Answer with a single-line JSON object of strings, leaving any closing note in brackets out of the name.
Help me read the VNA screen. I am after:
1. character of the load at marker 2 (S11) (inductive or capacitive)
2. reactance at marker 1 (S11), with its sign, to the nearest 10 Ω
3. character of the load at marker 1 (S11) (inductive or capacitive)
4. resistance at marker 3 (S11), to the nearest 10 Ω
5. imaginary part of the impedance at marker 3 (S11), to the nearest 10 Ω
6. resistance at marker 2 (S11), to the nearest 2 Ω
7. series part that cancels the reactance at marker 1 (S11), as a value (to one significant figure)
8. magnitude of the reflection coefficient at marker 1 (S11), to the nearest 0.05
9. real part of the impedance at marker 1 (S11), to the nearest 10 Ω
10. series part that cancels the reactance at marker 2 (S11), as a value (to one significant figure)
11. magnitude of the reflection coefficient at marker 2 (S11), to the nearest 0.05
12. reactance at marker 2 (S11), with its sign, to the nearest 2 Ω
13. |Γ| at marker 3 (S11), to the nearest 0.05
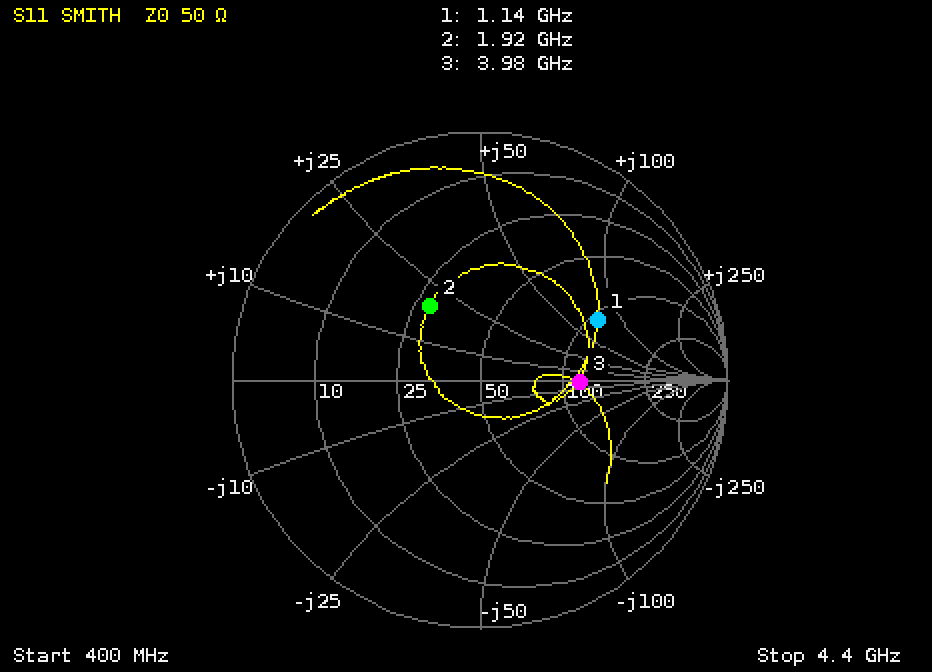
{"character of the load at marker 2 (S11)": "inductive", "reactance at marker 1 (S11), with its sign, to the nearest 10 Ω": "+70 Ω", "character of the load at marker 1 (S11)": "inductive", "resistance at marker 3 (S11), to the nearest 10 Ω": "120 Ω", "imaginary part of the impedance at marker 3 (S11), to the nearest 10 Ω": "0 Ω", "resistance at marker 2 (S11), to the nearest 2 Ω": "28 Ω", "series part that cancels the reactance at marker 1 (S11), as a value": "2 pF", "magnitude of the reflection coefficient at marker 1 (S11), to the nearest 0.05": "0.55", "real part of the impedance at marker 1 (S11), to the nearest 10 Ω": "110 Ω", "series part that cancels the reactance at marker 2 (S11), as a value": "4 pF", "magnitude of the reflection coefficient at marker 2 (S11), to the nearest 0.05": "0.35", "reactance at marker 2 (S11), with its sign, to the nearest 2 Ω": "+20 Ω", "|Γ| at marker 3 (S11), to the nearest 0.05": "0.40"}
